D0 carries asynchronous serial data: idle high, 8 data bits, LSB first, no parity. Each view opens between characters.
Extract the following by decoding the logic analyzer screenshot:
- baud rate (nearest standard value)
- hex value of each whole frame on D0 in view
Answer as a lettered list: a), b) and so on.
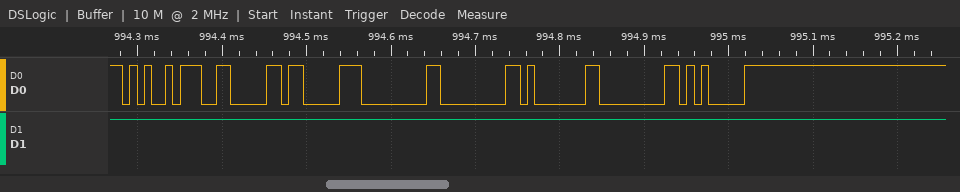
a) 115200 baud
b) A5, 06, 83, 00, 00, 01, 00, 05
